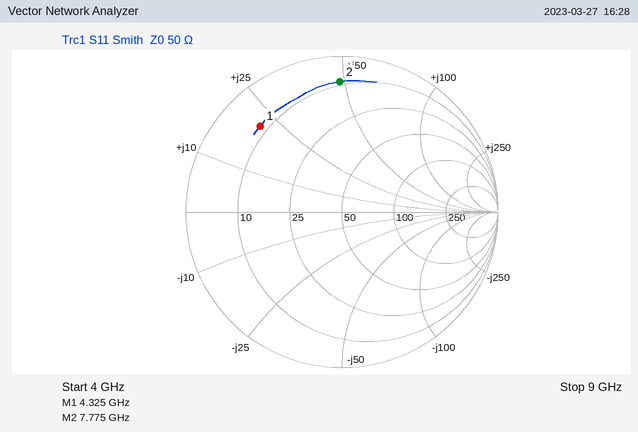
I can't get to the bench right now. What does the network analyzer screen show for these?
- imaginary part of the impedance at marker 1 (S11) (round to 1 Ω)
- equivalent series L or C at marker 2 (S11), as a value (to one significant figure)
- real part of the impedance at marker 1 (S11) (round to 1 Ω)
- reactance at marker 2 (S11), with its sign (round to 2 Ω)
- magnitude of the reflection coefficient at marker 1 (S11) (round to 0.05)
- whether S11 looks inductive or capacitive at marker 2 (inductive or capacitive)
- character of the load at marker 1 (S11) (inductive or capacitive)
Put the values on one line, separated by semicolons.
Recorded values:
+21 Ω; 1.0 nH; 8 Ω; +48 Ω; 0.75; inductive; inductive
